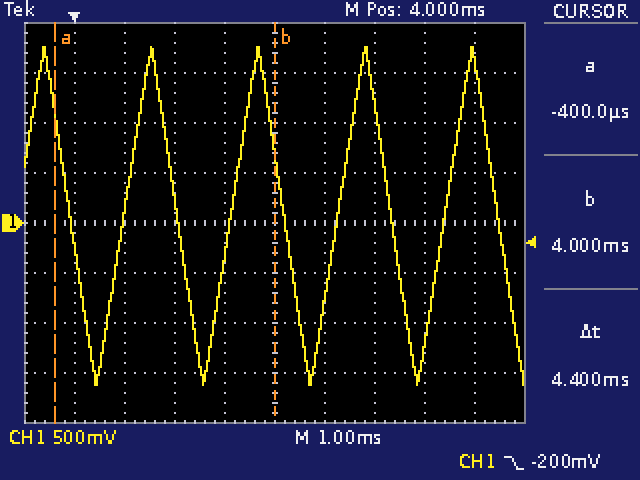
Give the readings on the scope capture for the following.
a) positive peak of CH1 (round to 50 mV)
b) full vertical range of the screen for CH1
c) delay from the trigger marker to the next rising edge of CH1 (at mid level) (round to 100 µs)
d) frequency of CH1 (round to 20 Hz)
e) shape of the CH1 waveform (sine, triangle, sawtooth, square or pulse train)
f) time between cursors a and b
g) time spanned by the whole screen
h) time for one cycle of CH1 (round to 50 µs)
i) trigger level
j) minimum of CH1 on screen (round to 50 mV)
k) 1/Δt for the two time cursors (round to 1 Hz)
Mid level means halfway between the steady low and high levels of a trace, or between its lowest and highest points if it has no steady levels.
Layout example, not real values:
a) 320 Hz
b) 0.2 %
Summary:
a) 1.75 V
b) 4 V
c) 1.0 ms
d) 460 Hz
e) triangle
f) 4.4 ms
g) 10 ms
h) 2.15 ms
i) -200 mV
j) -1.60 V
k) 227 Hz
